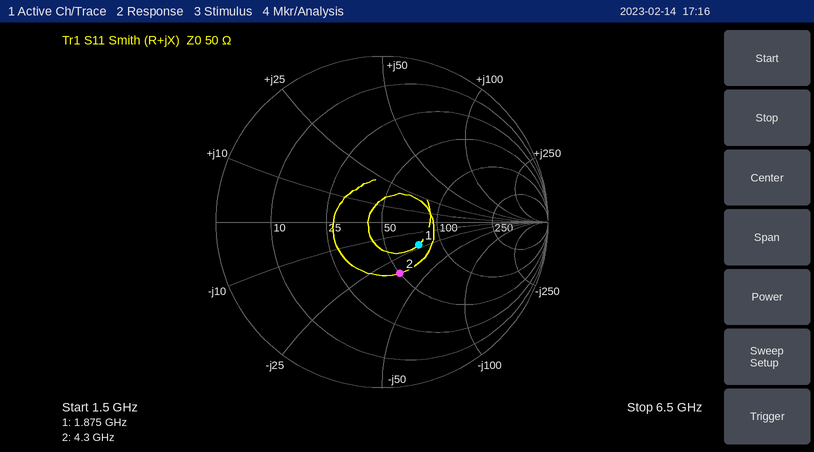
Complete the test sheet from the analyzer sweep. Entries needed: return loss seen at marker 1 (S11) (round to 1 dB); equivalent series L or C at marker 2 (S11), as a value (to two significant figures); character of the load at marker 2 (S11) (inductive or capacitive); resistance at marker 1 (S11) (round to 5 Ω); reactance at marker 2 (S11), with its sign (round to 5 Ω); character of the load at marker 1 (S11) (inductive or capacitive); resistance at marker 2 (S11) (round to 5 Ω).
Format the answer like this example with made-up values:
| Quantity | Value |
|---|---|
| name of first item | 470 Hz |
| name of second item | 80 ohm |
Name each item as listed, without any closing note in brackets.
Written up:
| Quantity | Value |
|---|---|
| return loss seen at marker 1 (S11) | 12 dB |
| equivalent series L or C at marker 2 (S11), as a value | 1.1 pF |
| character of the load at marker 2 (S11) | capacitive |
| resistance at marker 1 (S11) | 75 Ω |
| reactance at marker 2 (S11), with its sign | -35 Ω |
| character of the load at marker 1 (S11) | capacitive |
| resistance at marker 2 (S11) | 50 Ω |
